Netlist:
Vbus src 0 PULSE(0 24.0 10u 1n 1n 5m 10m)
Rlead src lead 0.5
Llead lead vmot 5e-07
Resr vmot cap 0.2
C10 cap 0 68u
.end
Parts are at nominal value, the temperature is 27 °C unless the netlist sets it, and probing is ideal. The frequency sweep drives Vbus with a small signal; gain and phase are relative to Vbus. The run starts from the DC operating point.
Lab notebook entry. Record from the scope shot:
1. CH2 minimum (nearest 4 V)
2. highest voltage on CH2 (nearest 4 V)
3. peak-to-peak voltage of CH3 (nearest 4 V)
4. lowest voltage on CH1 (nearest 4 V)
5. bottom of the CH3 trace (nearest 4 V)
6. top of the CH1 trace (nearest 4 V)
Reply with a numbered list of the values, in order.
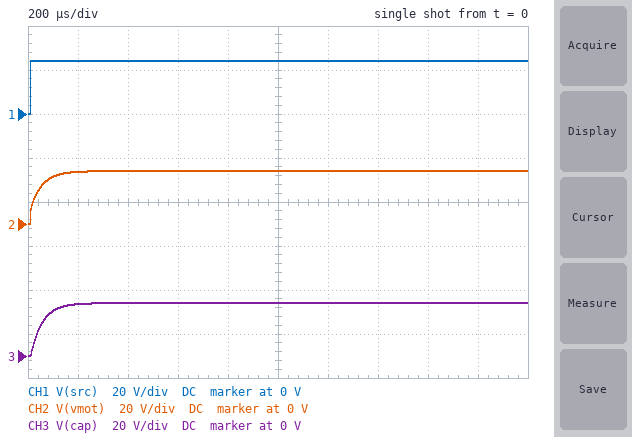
1. 0 V
2. 24 V
3. 24 V
4. 0 V
5. 0 V
6. 24 V
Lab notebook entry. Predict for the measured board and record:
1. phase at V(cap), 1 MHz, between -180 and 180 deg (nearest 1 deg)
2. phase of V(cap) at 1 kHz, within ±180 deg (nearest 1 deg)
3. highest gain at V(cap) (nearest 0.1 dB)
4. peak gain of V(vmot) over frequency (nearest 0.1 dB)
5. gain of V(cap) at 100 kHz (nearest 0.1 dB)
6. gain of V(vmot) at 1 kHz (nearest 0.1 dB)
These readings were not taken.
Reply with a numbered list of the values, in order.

1. -167 deg
2. -17 deg
3. 0 dB
4. 0 dB
5. -30.2 dB
6. -0.3 dB
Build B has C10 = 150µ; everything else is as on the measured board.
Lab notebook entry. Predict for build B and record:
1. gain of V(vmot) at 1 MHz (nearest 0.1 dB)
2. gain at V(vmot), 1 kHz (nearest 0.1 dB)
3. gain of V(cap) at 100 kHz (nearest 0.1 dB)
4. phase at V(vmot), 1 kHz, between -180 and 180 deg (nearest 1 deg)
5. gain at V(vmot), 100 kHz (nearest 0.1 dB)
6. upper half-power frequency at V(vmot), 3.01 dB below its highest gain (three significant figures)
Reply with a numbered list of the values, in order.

1. -24.1 dB
2. -1.4 dB
3. -37.1 dB
4. -23 deg
5. -11.6 dB
6. 1.67 kHz
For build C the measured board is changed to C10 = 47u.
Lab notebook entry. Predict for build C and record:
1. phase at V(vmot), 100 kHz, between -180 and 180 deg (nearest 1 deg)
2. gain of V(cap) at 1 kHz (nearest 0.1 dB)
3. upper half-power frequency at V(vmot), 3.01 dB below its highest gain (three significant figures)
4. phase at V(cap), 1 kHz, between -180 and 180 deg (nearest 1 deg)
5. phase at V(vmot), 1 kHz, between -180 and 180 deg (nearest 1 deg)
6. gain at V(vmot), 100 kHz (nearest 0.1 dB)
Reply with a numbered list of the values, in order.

1. -31 deg
2. -0.2 dB
3. 5.43 kHz
4. -12 deg
5. -8 deg
6. -11.4 dB
